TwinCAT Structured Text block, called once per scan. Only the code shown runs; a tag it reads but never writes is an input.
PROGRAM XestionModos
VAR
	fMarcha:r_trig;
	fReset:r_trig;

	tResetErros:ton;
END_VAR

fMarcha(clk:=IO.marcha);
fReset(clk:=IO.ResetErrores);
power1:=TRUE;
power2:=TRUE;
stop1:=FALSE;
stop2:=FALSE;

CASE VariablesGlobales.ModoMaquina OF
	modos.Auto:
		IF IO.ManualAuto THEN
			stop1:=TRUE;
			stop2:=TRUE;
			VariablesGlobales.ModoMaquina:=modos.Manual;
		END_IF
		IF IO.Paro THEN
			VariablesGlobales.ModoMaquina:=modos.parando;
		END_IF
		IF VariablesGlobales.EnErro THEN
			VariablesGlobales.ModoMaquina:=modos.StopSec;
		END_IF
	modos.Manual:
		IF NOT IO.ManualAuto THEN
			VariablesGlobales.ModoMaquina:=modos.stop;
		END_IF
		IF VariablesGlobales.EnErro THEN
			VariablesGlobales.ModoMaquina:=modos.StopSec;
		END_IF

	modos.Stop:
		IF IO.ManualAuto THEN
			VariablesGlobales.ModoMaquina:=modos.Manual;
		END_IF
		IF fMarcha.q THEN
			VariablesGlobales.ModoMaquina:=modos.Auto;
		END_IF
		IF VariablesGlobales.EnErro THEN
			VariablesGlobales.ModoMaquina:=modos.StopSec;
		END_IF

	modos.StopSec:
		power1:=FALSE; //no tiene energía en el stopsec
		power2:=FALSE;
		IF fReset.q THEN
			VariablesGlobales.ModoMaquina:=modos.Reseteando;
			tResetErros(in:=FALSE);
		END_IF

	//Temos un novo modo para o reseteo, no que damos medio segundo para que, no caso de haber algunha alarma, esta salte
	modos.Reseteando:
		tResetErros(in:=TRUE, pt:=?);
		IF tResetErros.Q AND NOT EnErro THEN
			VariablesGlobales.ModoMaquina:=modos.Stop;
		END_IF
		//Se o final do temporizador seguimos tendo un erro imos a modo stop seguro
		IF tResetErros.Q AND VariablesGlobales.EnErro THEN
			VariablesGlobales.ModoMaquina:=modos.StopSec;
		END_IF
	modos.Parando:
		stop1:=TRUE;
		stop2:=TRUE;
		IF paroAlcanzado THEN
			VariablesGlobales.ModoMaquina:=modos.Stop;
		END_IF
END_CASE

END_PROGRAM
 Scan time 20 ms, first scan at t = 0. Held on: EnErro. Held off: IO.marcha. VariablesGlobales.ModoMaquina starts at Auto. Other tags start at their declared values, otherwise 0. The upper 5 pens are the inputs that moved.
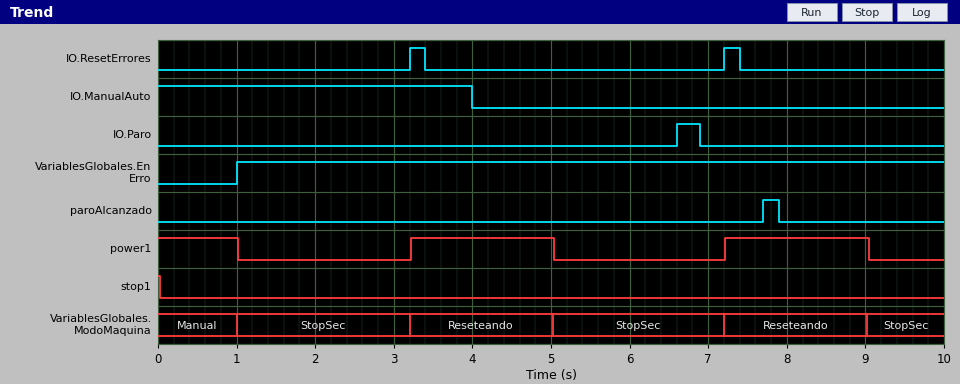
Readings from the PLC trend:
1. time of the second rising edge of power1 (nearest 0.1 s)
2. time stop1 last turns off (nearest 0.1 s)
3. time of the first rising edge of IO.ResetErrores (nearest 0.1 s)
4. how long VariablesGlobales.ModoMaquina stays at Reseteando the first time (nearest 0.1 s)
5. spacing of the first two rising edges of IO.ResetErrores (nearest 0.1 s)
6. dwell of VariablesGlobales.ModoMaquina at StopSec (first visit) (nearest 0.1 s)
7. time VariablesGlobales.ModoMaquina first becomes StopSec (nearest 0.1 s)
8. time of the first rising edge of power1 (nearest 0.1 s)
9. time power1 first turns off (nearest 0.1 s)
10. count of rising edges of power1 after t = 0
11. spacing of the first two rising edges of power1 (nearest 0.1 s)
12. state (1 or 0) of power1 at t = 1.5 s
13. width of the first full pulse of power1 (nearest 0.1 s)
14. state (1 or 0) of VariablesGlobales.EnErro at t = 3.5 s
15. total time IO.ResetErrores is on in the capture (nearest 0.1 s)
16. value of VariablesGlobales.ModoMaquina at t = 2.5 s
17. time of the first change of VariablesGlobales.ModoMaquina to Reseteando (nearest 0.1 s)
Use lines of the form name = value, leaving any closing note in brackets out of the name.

time of the second rising edge of power1 = 7.2 s
time stop1 last turns off = 0.0 s
time of the first rising edge of IO.ResetErrores = 3.2 s
how long VariablesGlobales.ModoMaquina stays at Reseteando the first time = 1.8 s
spacing of the first two rising edges of IO.ResetErrores = 4.0 s
dwell of VariablesGlobales.ModoMaquina at StopSec (first visit) = 2.2 s
time VariablesGlobales.ModoMaquina first becomes StopSec = 1.0 s
time of the first rising edge of power1 = 3.2 s
time power1 first turns off = 1.0 s
count of rising edges of power1 after t = 0 = 2
spacing of the first two rising edges of power1 = 4.0 s
state (1 or 0) of power1 at t = 1.5 s = 0
width of the first full pulse of power1 = 1.8 s
state (1 or 0) of VariablesGlobales.EnErro at t = 3.5 s = 1
total time IO.ResetErrores is on in the capture = 0.4 s
value of VariablesGlobales.ModoMaquina at t = 2.5 s = StopSec
time of the first change of VariablesGlobales.ModoMaquina to Reseteando = 3.2 s
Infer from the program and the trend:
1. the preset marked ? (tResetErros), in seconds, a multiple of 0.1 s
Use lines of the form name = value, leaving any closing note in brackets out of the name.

the preset marked ? (tResetErros), in seconds, a multiple of 0.1 s = 1.8 s
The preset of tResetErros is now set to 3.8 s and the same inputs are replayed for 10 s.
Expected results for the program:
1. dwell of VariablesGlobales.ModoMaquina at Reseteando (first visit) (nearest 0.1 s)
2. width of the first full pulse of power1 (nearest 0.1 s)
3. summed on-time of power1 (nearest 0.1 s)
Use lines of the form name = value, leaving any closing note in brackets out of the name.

dwell of VariablesGlobales.ModoMaquina at Reseteando (first visit) = 3.8 s
width of the first full pulse of power1 = 3.8 s
summed on-time of power1 = 7.6 s
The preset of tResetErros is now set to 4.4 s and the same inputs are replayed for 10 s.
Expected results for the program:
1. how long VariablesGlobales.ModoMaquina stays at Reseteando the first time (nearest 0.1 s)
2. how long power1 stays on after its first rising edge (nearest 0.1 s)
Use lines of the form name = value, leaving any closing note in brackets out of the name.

how long VariablesGlobales.ModoMaquina stays at Reseteando the first time = 4.4 s
how long power1 stays on after its first rising edge = 4.4 s
